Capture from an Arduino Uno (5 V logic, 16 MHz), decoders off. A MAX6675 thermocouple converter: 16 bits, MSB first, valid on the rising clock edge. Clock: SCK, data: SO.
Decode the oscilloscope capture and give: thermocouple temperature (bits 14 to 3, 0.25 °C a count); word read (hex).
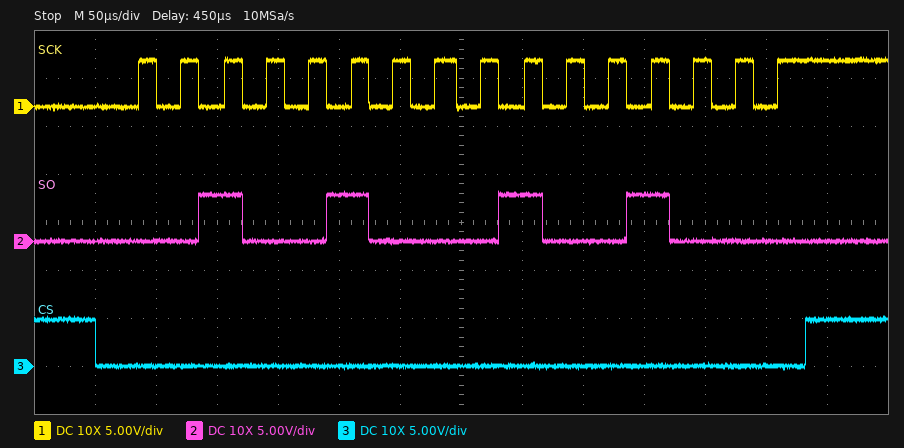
290.25 °C
0x2448
